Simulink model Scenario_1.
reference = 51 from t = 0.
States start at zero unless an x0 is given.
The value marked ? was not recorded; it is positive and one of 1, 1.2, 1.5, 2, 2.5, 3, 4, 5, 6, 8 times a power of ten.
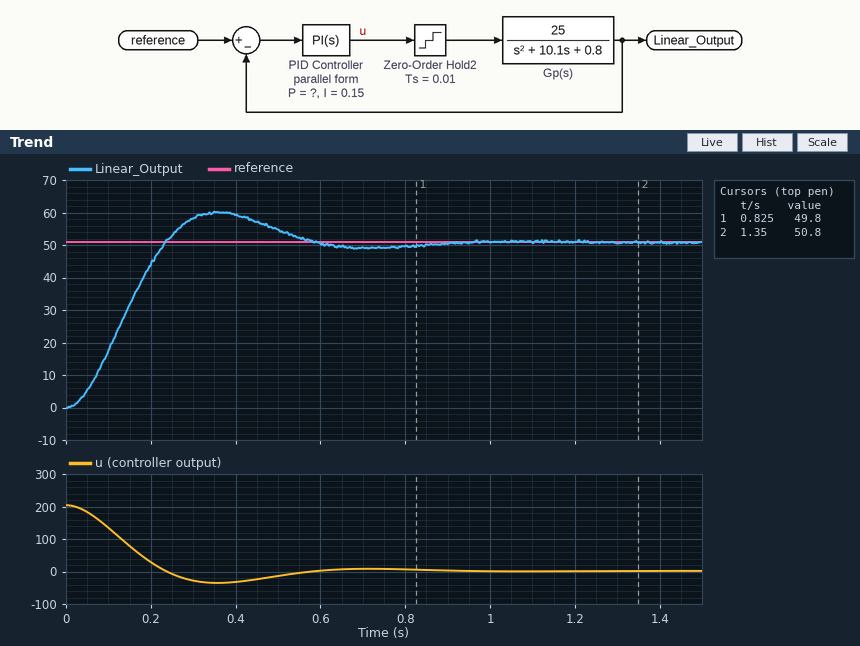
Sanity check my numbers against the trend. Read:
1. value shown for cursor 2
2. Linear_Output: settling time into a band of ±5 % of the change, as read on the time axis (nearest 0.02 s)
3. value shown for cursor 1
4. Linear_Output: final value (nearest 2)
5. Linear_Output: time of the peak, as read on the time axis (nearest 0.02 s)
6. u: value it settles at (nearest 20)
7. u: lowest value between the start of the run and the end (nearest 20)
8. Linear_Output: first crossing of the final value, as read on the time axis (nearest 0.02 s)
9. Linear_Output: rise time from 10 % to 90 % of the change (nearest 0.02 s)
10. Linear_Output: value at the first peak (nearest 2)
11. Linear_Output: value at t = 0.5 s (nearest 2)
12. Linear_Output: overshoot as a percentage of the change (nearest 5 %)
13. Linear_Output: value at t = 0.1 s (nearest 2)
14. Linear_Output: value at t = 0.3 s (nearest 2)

50.8
0.52 s
49.8
50
0.36 s
0
-40
0.24 s
0.16 s
60
54
20 %
18
58
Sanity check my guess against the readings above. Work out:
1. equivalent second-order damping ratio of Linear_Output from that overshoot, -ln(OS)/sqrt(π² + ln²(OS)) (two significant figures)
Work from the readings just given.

0.46
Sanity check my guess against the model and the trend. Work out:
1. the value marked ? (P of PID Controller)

4
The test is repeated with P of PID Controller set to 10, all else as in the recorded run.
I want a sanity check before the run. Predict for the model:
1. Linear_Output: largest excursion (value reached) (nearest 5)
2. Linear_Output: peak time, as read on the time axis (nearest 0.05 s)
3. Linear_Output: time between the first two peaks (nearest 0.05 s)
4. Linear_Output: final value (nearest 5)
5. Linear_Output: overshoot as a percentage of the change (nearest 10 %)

70
0.20 s
0.40 s
50
40 %
